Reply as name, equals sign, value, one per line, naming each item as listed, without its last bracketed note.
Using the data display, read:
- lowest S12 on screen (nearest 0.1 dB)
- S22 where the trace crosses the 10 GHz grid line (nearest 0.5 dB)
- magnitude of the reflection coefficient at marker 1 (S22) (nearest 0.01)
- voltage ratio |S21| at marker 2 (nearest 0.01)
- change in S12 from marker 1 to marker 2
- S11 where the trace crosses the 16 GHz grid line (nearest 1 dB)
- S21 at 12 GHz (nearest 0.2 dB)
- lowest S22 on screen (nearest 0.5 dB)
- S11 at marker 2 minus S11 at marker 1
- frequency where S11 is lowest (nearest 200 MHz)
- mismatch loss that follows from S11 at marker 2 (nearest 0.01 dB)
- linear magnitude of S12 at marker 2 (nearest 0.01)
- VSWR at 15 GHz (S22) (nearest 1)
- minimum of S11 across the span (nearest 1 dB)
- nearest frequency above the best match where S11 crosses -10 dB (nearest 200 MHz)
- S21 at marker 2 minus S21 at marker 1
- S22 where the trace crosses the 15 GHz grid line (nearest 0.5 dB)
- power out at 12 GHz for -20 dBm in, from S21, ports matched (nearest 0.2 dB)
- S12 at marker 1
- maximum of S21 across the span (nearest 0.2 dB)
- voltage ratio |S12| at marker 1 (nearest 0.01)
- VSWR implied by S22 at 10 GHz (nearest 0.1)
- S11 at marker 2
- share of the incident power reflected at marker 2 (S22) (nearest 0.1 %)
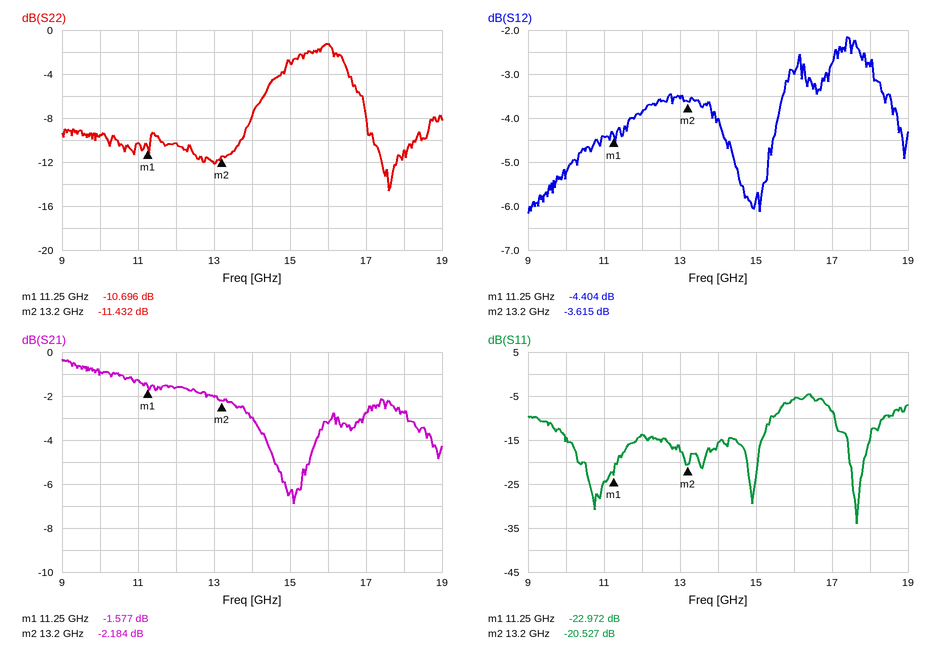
lowest S12 on screen = -6.2 dB
S22 where the trace crosses the 10 GHz grid line = -9.5 dB
magnitude of the reflection coefficient at marker 1 (S22) = 0.29
voltage ratio |S21| at marker 2 = 0.78
change in S12 from marker 1 to marker 2 = 0.789 dB
S11 where the trace crosses the 16 GHz grid line = -6 dB
S21 at 12 GHz = -1.6 dB
lowest S22 on screen = -14.5 dB
S11 at marker 2 minus S11 at marker 1 = 2.445 dB
frequency where S11 is lowest = 17.6 GHz
mismatch loss that follows from S11 at marker 2 = 0.04 dB
linear magnitude of S12 at marker 2 = 0.66
VSWR at 15 GHz (S22) = 6
minimum of S11 across the span = -34 dB
nearest frequency above the best match where S11 crosses -10 dB = 18.4 GHz
S21 at marker 2 minus S21 at marker 1 = -0.607 dB
S22 where the trace crosses the 15 GHz grid line = -3.0 dB
power out at 12 GHz for -20 dBm in, from S21, ports matched = -21.6 dBm
S12 at marker 1 = -4.404 dB
maximum of S21 across the span = -0.4 dB
voltage ratio |S12| at marker 1 = 0.60
VSWR implied by S22 at 10 GHz = 2.0
S11 at marker 2 = -20.527 dB
share of the incident power reflected at marker 2 (S22) = 7.2 %
